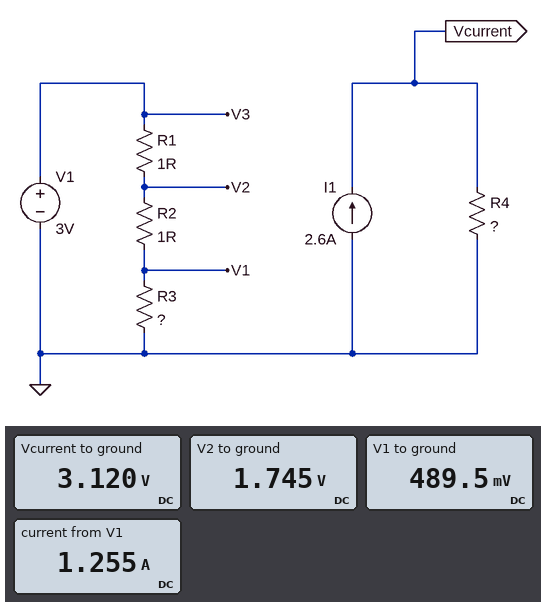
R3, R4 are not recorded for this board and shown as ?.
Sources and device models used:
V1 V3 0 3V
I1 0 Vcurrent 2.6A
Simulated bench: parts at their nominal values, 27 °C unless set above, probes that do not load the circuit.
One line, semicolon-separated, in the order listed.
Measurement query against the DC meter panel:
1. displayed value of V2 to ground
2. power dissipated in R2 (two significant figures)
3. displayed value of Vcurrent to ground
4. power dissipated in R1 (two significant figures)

1.745 V; 1.6 W; 3.120 V; 1.6 W
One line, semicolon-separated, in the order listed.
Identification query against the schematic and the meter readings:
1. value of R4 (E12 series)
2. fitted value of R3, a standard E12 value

1.2 Ω; 0.39 Ω
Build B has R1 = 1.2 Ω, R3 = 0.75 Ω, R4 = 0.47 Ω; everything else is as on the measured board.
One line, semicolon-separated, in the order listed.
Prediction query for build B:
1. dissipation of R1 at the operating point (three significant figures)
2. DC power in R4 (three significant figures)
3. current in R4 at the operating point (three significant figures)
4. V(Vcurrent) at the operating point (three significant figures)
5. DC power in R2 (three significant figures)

1.24 W; 3.18 W; 2.60 A; 1.22 V; 1.03 W
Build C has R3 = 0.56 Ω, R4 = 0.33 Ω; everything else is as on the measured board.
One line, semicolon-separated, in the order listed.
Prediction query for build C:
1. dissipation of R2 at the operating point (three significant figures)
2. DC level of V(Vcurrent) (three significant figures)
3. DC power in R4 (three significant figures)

1.37 W; 858 mV; 2.23 W
